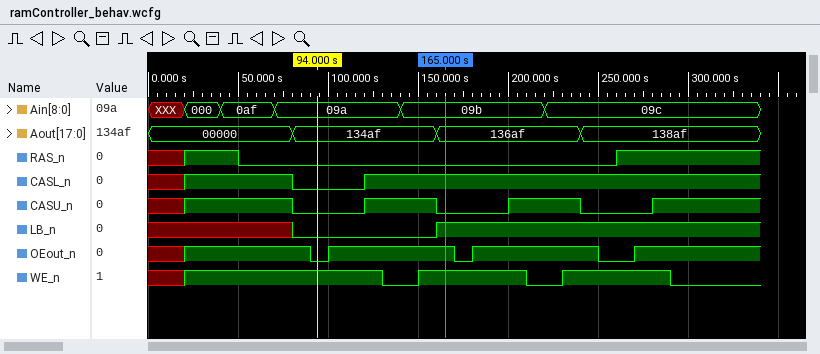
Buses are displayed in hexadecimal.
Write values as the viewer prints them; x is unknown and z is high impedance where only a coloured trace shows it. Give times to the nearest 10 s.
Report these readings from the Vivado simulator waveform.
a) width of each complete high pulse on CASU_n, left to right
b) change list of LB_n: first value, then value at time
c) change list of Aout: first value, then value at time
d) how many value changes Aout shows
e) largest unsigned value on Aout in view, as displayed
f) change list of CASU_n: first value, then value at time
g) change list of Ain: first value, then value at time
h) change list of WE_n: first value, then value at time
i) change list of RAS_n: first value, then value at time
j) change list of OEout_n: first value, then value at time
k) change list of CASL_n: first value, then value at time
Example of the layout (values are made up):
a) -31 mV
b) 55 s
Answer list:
a) 40 s, 40 s
b) x, 0 at 80 s, 1 at 160 s
c) 00000, 134af at 80 s, 136af at 160 s, 138af at 240 s
d) 3
e) 138af
f) x, 1 at 20 s, 0 at 80 s, 1 at 120 s, 0 at 160 s, 1 at 200 s, 0 at 240 s, 1 at 280 s
g) XXX, 000 at 20 s, 0af at 40 s, 09a at 70 s, 09b at 140 s, 09c at 220 s
h) x, 1 at 20 s, 0 at 130 s, 1 at 150 s, 0 at 210 s, 1 at 230 s, 0 at 290 s
i) x, 1 at 20 s, 0 at 50 s, 1 at 260 s
j) x, 1 at 20 s, 0 at 90 s, 1 at 100 s, 0 at 170 s, 1 at 180 s, 0 at 250 s, 1 at 270 s
k) x, 1 at 20 s, 0 at 80 s, 1 at 120 s
